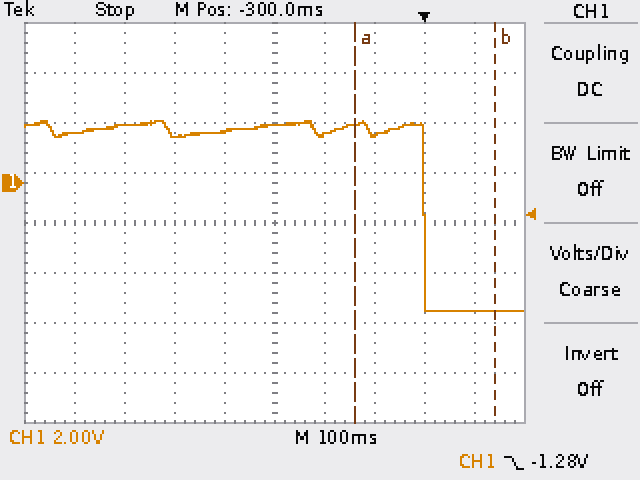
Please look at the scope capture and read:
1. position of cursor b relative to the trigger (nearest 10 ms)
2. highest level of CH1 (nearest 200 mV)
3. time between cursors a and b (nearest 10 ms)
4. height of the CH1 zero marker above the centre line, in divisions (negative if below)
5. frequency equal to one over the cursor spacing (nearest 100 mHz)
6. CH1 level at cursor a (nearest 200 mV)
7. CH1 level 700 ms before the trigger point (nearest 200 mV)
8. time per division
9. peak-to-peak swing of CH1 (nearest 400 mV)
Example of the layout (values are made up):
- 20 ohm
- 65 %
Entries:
- +140 ms
- 2.4 V
- 280 ms
- +0.8 div
- 3.6 Hz
- 2.4 V
- 2.0 V
- 100 ms
- 7.6 V
